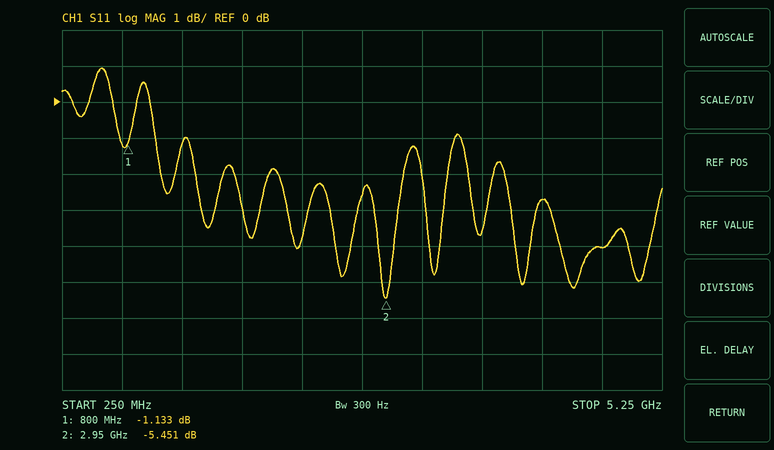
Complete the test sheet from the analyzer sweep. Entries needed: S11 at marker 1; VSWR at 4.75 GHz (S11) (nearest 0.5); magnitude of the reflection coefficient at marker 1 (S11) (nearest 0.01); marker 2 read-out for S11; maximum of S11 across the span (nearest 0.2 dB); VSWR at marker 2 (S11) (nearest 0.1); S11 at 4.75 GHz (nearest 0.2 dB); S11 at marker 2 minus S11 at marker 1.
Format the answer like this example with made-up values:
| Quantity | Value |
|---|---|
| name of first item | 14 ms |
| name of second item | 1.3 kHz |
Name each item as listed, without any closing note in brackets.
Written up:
| Quantity | Value |
|---|---|
| S11 at marker 1 | -1.133 dB |
| VSWR at 4.75 GHz (S11) | 4.5 |
| magnitude of the reflection coefficient at marker 1 (S11) | 0.88 |
| marker 2 read-out for S11 | -5.451 dB |
| maximum of S11 across the span | 1.0 dB |
| VSWR at marker 2 (S11) | 3.3 |
| S11 at 4.75 GHz | -4.0 dB |
| S11 at marker 2 minus S11 at marker 1 | -4.318 dB |
